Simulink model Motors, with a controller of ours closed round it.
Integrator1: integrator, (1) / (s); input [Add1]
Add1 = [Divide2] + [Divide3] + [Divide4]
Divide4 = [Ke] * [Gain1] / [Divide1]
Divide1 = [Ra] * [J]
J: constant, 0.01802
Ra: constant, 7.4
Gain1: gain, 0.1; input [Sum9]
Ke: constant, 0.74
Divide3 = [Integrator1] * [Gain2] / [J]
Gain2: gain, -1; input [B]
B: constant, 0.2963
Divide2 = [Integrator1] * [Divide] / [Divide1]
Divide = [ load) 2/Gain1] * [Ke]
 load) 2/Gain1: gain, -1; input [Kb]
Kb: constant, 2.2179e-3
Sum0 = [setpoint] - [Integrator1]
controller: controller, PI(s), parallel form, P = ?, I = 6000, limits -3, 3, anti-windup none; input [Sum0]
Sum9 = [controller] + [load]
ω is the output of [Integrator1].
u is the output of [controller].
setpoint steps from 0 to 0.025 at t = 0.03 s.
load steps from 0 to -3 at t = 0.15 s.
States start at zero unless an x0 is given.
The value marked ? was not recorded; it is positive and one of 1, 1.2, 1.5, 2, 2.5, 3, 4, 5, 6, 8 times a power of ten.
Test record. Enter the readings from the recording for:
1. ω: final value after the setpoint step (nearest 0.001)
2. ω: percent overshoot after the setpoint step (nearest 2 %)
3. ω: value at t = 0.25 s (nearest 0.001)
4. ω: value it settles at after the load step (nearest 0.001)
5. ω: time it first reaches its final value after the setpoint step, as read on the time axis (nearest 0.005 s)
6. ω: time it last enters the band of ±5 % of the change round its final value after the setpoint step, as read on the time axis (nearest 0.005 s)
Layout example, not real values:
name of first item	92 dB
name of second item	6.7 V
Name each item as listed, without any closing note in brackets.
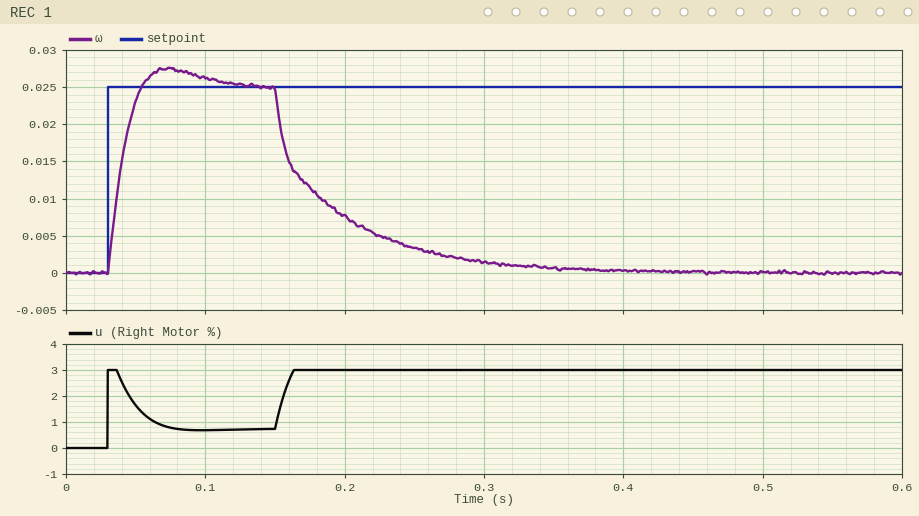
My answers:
ω: final value after the setpoint step	0.025
ω: percent overshoot after the setpoint step	10 %
ω: value at t = 0.25 s	0.003
ω: value it settles at after the load step	0.000
ω: time it first reaches its final value after the setpoint step, as read on the time axis	0.055 s
ω: time it last enters the band of ±5 % of the change round its final value after the setpoint step, as read on the time axis	0.100 s
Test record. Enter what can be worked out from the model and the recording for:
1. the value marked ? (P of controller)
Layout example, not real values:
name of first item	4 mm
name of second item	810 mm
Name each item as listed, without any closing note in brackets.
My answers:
the value marked ?	150
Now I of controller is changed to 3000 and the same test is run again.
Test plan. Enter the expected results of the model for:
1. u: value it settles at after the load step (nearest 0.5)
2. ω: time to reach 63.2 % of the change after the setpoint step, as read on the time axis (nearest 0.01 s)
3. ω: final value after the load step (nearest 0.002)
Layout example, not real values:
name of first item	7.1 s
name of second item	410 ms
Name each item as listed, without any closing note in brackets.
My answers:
u: value it settles at after the load step	3.0
ω: time to reach 63.2 % of the change after the setpoint step, as read on the time axis	0.04 s
ω: final value after the load step	0.000
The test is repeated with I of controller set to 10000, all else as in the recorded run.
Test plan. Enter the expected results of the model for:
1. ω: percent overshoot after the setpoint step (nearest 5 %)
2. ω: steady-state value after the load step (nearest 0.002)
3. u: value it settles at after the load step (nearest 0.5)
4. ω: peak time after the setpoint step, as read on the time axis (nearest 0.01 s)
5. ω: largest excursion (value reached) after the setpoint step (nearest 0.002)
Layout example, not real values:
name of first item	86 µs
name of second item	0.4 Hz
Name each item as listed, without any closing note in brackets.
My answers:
ω: percent overshoot after the setpoint step	20 %
ω: steady-state value after the load step	0.000
u: value it settles at after the load step	3.0
ω: peak time after the setpoint step, as read on the time axis	0.06 s
ω: largest excursion (value reached) after the setpoint step	0.030
